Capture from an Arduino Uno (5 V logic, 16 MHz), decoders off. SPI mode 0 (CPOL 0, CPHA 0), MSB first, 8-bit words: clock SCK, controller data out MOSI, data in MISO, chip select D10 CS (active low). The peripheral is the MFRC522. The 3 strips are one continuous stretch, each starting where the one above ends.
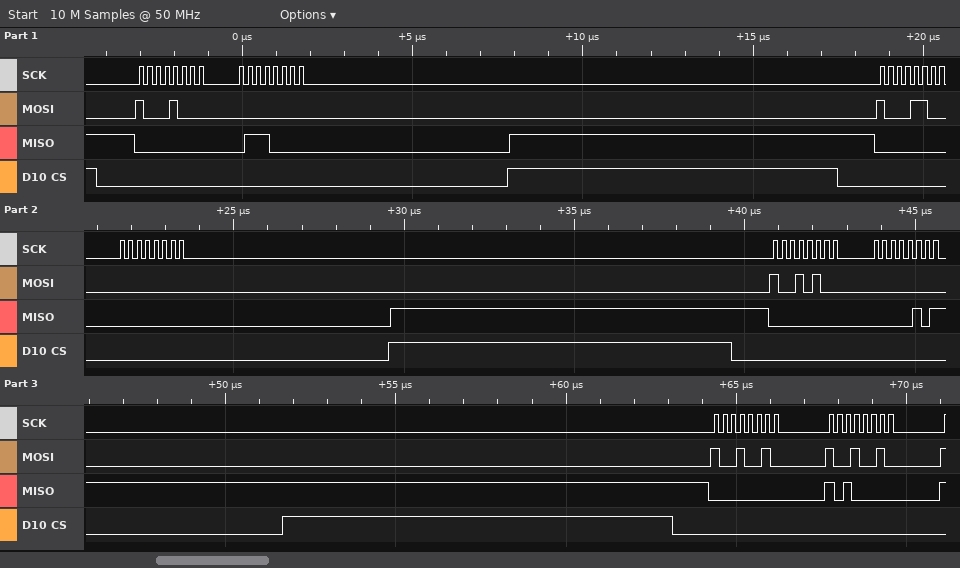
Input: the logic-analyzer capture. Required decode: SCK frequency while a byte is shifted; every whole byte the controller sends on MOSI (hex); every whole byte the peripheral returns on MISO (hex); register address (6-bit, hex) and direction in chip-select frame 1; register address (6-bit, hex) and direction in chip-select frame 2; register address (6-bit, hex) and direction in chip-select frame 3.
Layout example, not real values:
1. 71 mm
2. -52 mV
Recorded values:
1. 4 MHz
2. 0x88 0x00 0x8C 0x00 0x94 0x00 0x92 0x92
3. 0x00 0x70 0x00 0x00 0x00 0x05 0x00 0xA0
4. 0x04 read
5. 0x06 read
6. 0x0A read
